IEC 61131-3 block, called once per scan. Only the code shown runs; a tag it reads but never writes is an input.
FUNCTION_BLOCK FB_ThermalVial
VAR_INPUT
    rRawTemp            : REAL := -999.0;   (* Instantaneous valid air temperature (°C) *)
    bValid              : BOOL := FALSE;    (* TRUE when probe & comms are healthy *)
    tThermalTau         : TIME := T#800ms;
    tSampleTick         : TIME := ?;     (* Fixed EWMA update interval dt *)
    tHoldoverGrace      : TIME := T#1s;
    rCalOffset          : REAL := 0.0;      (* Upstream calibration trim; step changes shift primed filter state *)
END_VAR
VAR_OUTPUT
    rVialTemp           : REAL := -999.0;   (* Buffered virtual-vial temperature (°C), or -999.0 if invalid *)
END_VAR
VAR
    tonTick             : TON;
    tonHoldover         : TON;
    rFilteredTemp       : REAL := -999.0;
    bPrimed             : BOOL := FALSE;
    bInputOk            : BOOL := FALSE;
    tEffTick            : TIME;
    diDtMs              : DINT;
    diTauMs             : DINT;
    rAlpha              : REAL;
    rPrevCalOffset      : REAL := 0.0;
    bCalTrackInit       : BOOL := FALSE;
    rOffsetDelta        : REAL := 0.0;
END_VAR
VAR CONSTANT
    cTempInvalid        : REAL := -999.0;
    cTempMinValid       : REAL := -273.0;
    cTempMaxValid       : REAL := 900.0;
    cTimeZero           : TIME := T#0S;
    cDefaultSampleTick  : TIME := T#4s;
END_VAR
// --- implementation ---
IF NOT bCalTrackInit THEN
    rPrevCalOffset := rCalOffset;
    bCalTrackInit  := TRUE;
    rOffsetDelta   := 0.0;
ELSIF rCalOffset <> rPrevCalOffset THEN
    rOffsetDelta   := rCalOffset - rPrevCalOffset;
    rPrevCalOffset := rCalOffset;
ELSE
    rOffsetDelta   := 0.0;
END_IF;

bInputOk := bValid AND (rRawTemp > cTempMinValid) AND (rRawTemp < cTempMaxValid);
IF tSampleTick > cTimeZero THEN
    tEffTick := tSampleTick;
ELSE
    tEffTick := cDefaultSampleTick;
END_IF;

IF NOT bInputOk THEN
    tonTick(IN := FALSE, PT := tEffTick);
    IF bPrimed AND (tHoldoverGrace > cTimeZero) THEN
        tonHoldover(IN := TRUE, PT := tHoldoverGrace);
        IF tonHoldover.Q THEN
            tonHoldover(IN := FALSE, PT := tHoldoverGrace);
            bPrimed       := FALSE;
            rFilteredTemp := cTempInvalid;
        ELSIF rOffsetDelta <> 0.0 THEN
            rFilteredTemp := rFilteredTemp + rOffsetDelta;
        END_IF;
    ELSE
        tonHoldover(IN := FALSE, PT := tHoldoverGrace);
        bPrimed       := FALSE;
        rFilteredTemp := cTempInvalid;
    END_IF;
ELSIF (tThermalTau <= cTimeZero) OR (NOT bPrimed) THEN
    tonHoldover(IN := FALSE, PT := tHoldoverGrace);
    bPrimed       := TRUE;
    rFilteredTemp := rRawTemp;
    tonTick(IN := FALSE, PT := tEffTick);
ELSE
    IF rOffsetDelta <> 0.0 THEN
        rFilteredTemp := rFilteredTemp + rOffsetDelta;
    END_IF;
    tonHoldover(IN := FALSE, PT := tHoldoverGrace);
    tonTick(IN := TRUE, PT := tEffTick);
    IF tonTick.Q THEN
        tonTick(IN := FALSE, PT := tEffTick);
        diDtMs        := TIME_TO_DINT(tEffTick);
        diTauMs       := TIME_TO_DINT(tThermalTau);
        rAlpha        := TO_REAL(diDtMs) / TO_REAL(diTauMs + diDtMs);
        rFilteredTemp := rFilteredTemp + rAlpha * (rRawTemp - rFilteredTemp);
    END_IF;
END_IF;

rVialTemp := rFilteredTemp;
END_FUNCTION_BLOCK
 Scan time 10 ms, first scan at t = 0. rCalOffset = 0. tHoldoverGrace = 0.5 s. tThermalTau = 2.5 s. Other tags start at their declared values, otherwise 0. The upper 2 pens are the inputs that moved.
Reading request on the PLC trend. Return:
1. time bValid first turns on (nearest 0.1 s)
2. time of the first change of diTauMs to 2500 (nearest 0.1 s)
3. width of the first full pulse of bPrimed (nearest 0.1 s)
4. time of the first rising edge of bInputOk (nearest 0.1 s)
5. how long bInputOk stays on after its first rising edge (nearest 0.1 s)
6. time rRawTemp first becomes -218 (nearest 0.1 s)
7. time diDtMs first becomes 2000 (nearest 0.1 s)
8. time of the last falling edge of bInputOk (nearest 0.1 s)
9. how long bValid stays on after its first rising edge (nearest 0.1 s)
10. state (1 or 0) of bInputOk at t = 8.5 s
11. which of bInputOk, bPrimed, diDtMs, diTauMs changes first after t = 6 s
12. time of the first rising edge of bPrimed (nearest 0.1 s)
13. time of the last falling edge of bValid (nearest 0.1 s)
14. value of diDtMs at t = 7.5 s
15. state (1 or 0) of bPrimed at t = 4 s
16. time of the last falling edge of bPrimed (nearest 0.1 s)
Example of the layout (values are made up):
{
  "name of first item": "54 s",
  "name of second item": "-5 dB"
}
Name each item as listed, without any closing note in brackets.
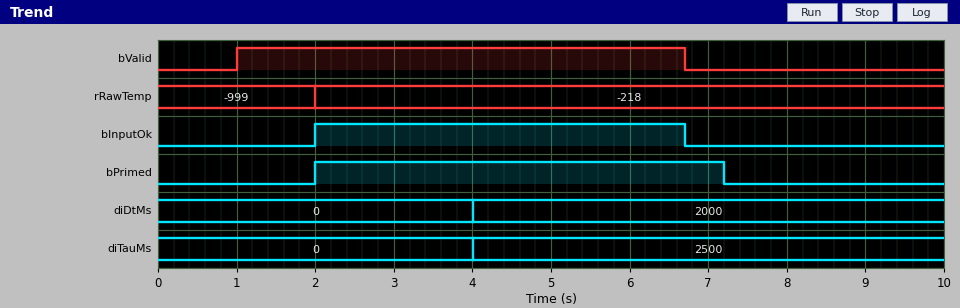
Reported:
{
  "time bValid first turns on": "1.0 s",
  "time of the first change of diTauMs to 2500": "4.0 s",
  "width of the first full pulse of bPrimed": "5.2 s",
  "time of the first rising edge of bInputOk": "2.0 s",
  "how long bInputOk stays on after its first rising edge": "4.7 s",
  "time rRawTemp first becomes -218": "2.0 s",
  "time diDtMs first becomes 2000": "4.0 s",
  "time of the last falling edge of bInputOk": "6.7 s",
  "how long bValid stays on after its first rising edge": "5.7 s",
  "state (1 or 0) of bInputOk at t = 8.5 s": "0",
  "which of bInputOk, bPrimed, diDtMs, diTauMs changes first after t = 6 s": "bInputOk",
  "time of the first rising edge of bPrimed": "2.0 s",
  "time of the last falling edge of bValid": "6.7 s",
  "value of diDtMs at t = 7.5 s": "2000",
  "state (1 or 0) of bPrimed at t = 4 s": "1",
  "time of the last falling edge of bPrimed": "7.2 s"
}
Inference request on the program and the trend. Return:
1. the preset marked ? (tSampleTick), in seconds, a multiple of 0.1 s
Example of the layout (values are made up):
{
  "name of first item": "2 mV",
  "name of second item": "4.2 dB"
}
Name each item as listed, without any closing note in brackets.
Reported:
{
  "the preset marked ? (tSampleTick), in seconds, a multiple of 0.1 s": "2.0 s"
}
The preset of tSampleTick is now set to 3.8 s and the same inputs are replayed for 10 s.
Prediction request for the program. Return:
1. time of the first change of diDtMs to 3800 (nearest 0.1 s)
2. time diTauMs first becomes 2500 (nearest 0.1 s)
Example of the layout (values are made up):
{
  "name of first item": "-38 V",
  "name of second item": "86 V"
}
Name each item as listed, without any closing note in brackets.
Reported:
{
  "time of the first change of diDtMs to 3800": "5.8 s",
  "time diTauMs first becomes 2500": "5.8 s"
}
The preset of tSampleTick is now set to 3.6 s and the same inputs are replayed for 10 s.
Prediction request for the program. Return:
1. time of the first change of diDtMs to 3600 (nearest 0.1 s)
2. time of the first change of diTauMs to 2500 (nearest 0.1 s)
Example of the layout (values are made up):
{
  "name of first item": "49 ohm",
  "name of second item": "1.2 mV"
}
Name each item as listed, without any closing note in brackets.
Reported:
{
  "time of the first change of diDtMs to 3600": "5.6 s",
  "time of the first change of diTauMs to 2500": "5.6 s"
}
